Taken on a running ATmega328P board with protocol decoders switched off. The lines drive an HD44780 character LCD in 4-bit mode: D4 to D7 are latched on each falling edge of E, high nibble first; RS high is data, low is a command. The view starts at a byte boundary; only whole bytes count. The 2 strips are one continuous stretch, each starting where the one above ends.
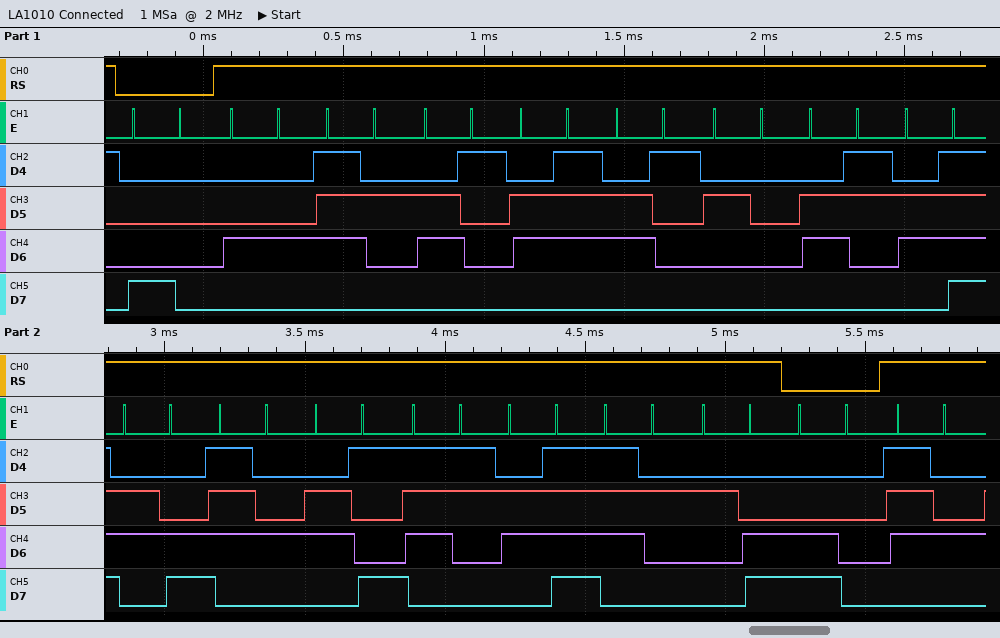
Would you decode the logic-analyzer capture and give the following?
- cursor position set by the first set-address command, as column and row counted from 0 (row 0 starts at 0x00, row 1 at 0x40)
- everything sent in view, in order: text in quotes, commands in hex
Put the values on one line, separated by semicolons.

column 0, row 0; 0x80 "Draga coltisor," 0xC0 "t"
